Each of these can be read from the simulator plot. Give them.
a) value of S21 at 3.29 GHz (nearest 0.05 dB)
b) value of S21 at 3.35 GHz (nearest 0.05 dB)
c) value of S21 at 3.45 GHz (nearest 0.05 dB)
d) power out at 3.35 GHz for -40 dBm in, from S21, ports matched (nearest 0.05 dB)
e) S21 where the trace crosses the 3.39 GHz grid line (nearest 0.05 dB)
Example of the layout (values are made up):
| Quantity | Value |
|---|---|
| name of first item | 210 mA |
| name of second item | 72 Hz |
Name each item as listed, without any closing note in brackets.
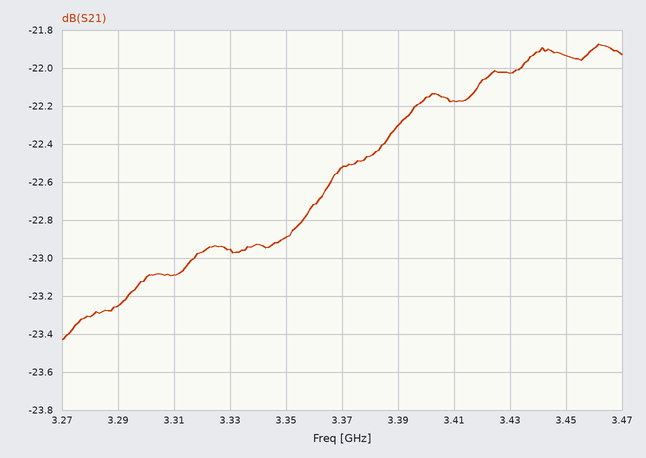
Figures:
| Quantity | Value |
|---|---|
| value of S21 at 3.29 GHz | -23.25 dB |
| value of S21 at 3.35 GHz | -22.90 dB |
| value of S21 at 3.45 GHz | -21.95 dB |
| power out at 3.35 GHz for -40 dBm in, from S21, ports matched | -62.90 dBm |
| S21 where the trace crosses the 3.39 GHz grid line | -22.30 dB |
